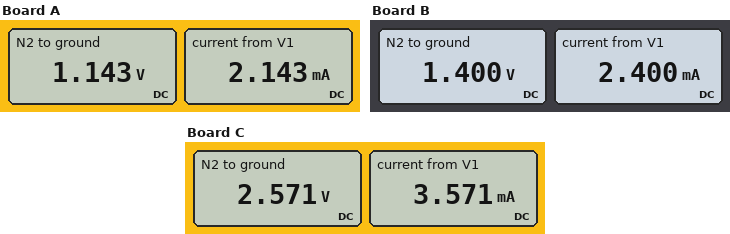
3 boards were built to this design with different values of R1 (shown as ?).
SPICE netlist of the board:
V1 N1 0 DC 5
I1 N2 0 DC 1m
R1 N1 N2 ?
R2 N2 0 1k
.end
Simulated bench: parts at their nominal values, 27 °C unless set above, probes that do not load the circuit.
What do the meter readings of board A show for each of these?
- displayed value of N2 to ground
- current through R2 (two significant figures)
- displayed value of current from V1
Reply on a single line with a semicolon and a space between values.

1.143 V; 1.1 mA; 2.143 mA
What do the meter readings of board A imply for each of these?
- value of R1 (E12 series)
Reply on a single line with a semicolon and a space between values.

1.8 kΩ
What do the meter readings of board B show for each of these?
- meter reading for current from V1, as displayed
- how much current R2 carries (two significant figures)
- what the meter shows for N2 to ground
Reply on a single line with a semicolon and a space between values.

2.400 mA; 1.4 mA; 1.400 V
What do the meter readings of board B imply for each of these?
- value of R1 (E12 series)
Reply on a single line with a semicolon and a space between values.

1.5 kΩ
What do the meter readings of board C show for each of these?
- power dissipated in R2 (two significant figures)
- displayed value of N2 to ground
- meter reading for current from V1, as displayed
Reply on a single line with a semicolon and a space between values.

6.6 mW; 2.571 V; 3.571 mA
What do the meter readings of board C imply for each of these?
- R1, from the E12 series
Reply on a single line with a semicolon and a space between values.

680 Ω
